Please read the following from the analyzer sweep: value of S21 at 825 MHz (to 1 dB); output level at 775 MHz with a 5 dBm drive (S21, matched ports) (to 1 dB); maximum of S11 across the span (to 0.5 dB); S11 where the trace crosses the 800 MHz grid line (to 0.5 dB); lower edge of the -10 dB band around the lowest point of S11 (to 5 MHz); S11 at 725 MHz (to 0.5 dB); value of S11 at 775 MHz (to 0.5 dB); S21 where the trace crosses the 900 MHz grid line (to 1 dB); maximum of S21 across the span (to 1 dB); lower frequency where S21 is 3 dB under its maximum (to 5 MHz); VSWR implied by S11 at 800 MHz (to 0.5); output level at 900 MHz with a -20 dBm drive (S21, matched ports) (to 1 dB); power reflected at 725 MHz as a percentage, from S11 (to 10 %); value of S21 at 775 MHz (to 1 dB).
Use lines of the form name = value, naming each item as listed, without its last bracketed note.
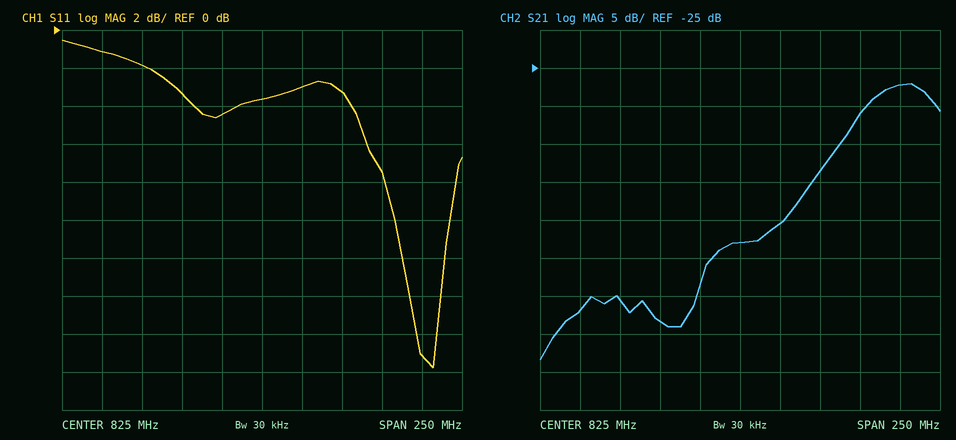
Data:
value of S21 at 825 MHz = -48 dB
output level at 775 MHz with a 5 dBm drive (S21, matched ports) = -53 dBm
maximum of S11 across the span = -0.5 dB
S11 where the trace crosses the 800 MHz grid line = -4.5 dB
lower edge of the -10 dB band around the lowest point of S11 = 910 MHz
S11 at 725 MHz = -1.0 dB
value of S11 at 775 MHz = -3.5 dB
S21 where the trace crosses the 900 MHz grid line = -31 dB
maximum of S21 across the span = -27 dB
lower frequency where S21 is 3 dB under its maximum = 905 MHz
VSWR implied by S11 at 800 MHz = 4.0
output level at 900 MHz with a -20 dBm drive (S21, matched ports) = -51 dBm
power reflected at 725 MHz as a percentage, from S11 = 80 %
value of S21 at 775 MHz = -58 dB
